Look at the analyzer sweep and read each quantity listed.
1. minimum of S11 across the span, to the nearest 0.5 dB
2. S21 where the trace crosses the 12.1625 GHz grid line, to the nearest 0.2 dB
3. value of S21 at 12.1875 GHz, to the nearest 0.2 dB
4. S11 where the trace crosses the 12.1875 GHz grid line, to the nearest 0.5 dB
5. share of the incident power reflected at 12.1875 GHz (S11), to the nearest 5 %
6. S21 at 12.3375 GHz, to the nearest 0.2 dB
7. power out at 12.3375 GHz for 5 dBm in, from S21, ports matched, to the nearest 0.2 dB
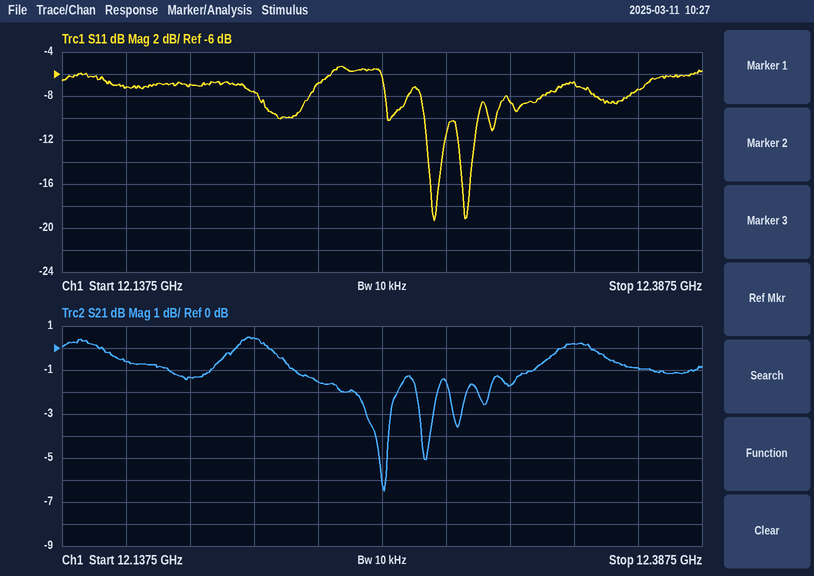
-19.5 dB
-0.6 dB
-1.4 dB
-7.0 dB
20 %
0.2 dB
5.2 dBm
